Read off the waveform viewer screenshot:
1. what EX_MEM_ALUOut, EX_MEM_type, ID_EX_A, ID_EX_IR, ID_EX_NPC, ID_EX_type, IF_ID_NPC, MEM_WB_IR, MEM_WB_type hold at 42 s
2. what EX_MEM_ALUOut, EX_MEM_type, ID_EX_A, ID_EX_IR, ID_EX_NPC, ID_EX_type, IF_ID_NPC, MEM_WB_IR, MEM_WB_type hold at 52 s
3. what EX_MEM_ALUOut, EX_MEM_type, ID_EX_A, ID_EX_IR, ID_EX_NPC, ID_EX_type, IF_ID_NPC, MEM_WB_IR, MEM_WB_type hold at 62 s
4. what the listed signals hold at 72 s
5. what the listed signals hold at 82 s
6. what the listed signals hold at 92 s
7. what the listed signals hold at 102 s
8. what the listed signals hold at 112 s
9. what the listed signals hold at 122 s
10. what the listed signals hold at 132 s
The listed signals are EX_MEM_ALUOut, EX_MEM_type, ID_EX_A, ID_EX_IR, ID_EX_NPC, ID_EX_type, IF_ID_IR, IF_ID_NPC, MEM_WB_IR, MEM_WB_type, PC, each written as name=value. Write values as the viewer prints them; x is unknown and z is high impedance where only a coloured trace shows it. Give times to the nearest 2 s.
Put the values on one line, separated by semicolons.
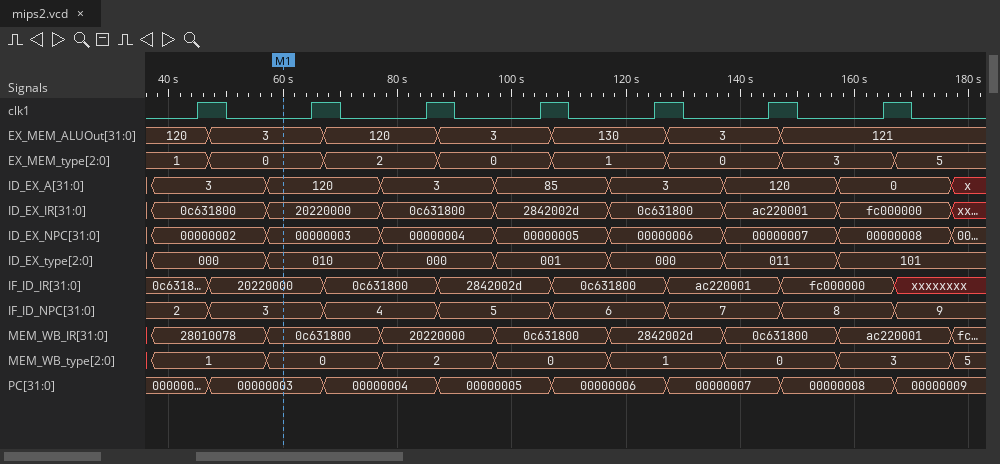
EX_MEM_ALUOut=120, EX_MEM_type=1, ID_EX_A=3, ID_EX_IR=0c631800, ID_EX_NPC=00000002, ID_EX_type=000, IF_ID_NPC=2, MEM_WB_IR=28010078, MEM_WB_type=1; EX_MEM_ALUOut=3, EX_MEM_type=0, ID_EX_A=3, ID_EX_IR=0c631800, ID_EX_NPC=00000002, ID_EX_type=000, IF_ID_NPC=3, MEM_WB_IR=28010078, MEM_WB_type=1; EX_MEM_ALUOut=3, EX_MEM_type=0, ID_EX_A=120, ID_EX_IR=20220000, ID_EX_NPC=00000003, ID_EX_type=010, IF_ID_NPC=3, MEM_WB_IR=0c631800, MEM_WB_type=0; EX_MEM_ALUOut=120, EX_MEM_type=2, ID_EX_A=120, ID_EX_IR=20220000, ID_EX_NPC=00000003, ID_EX_type=010, IF_ID_IR=0c631800, IF_ID_NPC=4, MEM_WB_IR=0c631800, MEM_WB_type=0, PC=00000004; EX_MEM_ALUOut=120, EX_MEM_type=2, ID_EX_A=3, ID_EX_IR=0c631800, ID_EX_NPC=00000004, ID_EX_type=000, IF_ID_IR=0c631800, IF_ID_NPC=4, MEM_WB_IR=20220000, MEM_WB_type=2, PC=00000004; EX_MEM_ALUOut=3, EX_MEM_type=0, ID_EX_A=3, ID_EX_IR=0c631800, ID_EX_NPC=00000004, ID_EX_type=000, IF_ID_IR=2842002d, IF_ID_NPC=5, MEM_WB_IR=20220000, MEM_WB_type=2, PC=00000005; EX_MEM_ALUOut=3, EX_MEM_type=0, ID_EX_A=85, ID_EX_IR=2842002d, ID_EX_NPC=00000005, ID_EX_type=001, IF_ID_IR=2842002d, IF_ID_NPC=5, MEM_WB_IR=0c631800, MEM_WB_type=0, PC=00000005; EX_MEM_ALUOut=130, EX_MEM_type=1, ID_EX_A=85, ID_EX_IR=2842002d, ID_EX_NPC=00000005, ID_EX_type=001, IF_ID_IR=0c631800, IF_ID_NPC=6, MEM_WB_IR=0c631800, MEM_WB_type=0, PC=00000006; EX_MEM_ALUOut=130, EX_MEM_type=1, ID_EX_A=3, ID_EX_IR=0c631800, ID_EX_NPC=00000006, ID_EX_type=000, IF_ID_IR=0c631800, IF_ID_NPC=6, MEM_WB_IR=2842002d, MEM_WB_type=1, PC=00000006; EX_MEM_ALUOut=3, EX_MEM_type=0, ID_EX_A=3, ID_EX_IR=0c631800, ID_EX_NPC=00000006, ID_EX_type=000, IF_ID_IR=ac220001, IF_ID_NPC=7, MEM_WB_IR=2842002d, MEM_WB_type=1, PC=00000007
